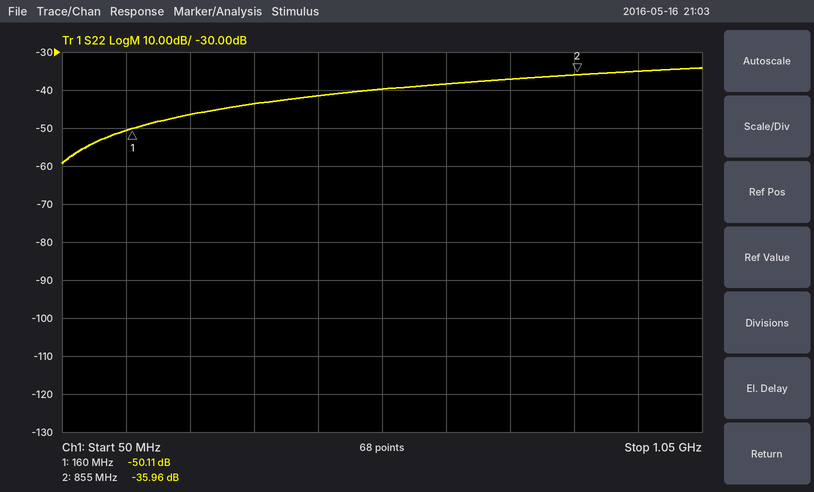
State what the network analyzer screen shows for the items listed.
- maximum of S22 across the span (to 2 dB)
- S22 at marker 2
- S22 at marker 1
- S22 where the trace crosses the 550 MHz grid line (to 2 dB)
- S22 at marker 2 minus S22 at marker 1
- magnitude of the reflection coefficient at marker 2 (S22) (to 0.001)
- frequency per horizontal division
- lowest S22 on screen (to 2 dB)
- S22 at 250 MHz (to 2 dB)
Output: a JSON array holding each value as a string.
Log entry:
["-34 dB", "-35.96 dB", "-50.11 dB", "-40 dB", "14.15 dB", "0.016", "100 MHz", "-60 dB", "-46 dB"]
